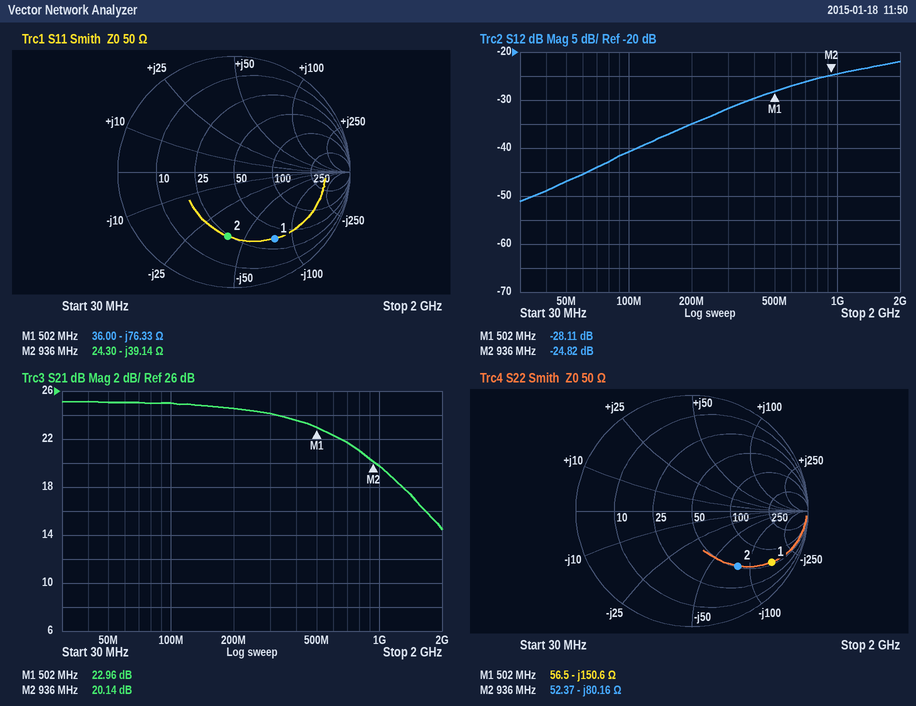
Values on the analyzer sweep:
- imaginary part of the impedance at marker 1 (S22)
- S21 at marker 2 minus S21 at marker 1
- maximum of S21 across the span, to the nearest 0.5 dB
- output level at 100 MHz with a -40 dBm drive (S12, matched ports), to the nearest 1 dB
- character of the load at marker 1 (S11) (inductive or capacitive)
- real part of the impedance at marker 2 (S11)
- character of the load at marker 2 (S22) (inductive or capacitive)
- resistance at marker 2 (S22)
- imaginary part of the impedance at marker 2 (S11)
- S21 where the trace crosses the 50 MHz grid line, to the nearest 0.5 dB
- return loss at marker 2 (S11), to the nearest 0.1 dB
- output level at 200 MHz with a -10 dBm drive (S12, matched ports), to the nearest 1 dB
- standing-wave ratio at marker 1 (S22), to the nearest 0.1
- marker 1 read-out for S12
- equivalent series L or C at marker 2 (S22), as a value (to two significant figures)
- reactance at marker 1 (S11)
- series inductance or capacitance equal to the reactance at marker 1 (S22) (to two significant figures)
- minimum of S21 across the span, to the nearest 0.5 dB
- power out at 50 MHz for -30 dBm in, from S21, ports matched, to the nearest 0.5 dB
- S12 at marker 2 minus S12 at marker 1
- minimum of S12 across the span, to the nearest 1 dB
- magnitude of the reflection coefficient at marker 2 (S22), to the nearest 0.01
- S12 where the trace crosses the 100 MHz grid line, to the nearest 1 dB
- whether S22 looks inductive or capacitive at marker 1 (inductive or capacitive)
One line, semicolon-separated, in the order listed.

-150.6 Ω; -2.82 dB; 25.0 dB; -81 dBm; capacitive; 24.30 Ω; capacitive; 52.37 Ω; -39.14 Ω; 25.0 dB; 5.1 dB; -45 dBm; 9.9; -28.11 dB; 2.1 pF; -76.33 Ω; 2.1 pF; 14.5 dB; -5.0 dBm; 3.29 dB; -51 dB; 0.62; -41 dB; capacitive
